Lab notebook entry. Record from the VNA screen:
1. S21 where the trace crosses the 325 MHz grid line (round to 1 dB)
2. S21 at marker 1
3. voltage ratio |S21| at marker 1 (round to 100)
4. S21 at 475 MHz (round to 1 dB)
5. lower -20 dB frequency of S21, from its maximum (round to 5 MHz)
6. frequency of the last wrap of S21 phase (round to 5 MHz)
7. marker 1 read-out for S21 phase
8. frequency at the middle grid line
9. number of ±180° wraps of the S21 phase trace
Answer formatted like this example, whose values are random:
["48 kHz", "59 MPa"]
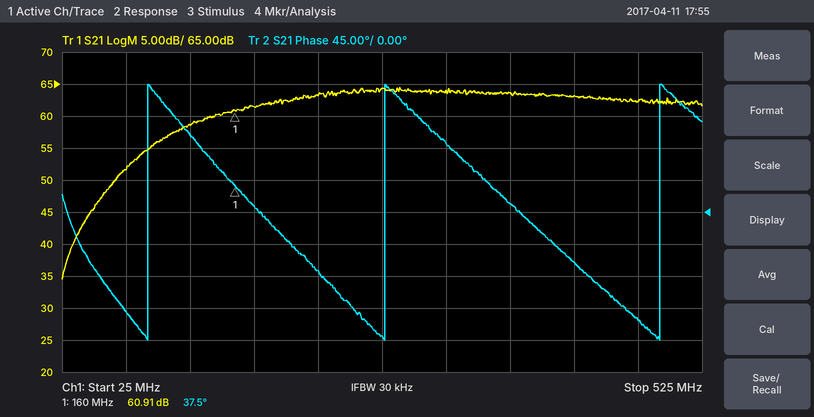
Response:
["64 dB", "60.91 dB", "1100", "62 dB", "45 MHz", "490 MHz", "37.5°", "275 MHz", "3"]
